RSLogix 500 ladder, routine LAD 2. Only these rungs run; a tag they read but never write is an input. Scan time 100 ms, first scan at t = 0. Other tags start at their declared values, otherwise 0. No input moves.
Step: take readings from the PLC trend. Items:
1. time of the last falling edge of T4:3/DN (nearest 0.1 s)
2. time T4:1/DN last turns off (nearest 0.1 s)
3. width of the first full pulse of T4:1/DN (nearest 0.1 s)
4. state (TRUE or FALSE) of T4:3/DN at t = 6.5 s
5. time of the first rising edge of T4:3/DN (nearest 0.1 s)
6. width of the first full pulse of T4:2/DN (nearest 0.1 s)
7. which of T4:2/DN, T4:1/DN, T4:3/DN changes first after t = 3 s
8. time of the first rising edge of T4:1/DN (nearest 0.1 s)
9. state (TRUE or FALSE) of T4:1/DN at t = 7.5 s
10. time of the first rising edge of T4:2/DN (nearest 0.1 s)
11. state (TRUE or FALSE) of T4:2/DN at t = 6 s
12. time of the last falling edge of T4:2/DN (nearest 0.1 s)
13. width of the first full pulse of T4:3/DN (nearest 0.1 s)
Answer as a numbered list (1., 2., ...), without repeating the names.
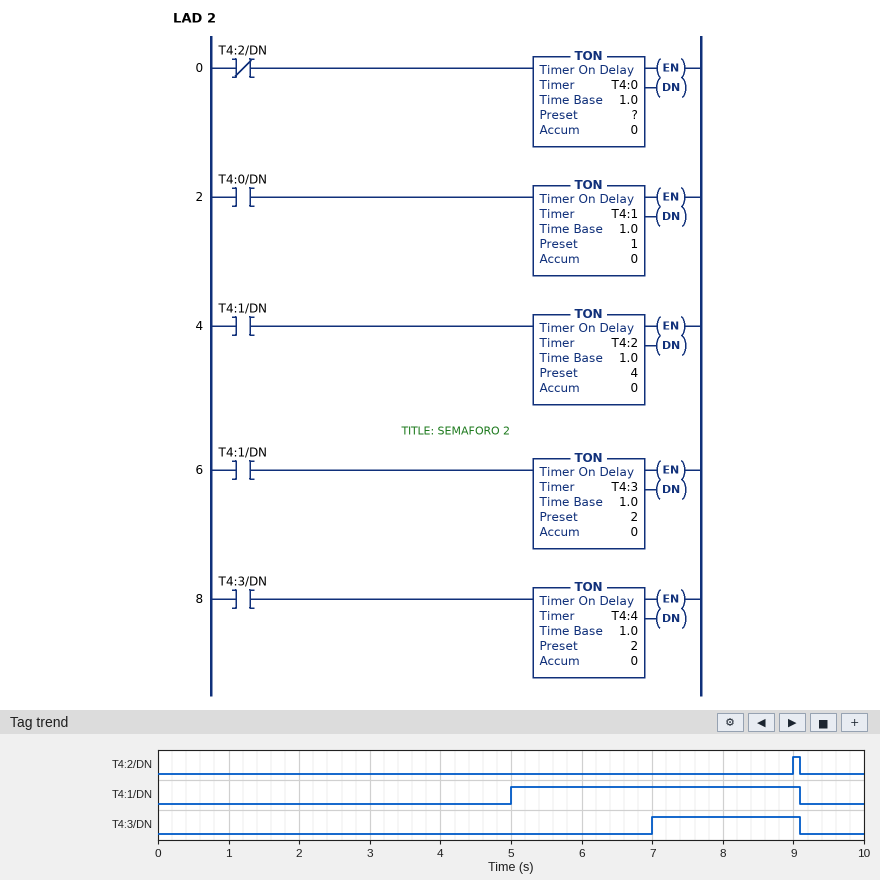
1. 9.1 s
2. 9.1 s
3. 4.1 s
4. FALSE
5. 7.0 s
6. 0.1 s
7. T4:1/DN
8. 5.0 s
9. TRUE
10. 9.0 s
11. FALSE
12. 9.1 s
13. 2.1 s
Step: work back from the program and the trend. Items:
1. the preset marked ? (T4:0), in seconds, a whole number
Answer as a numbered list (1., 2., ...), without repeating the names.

1. 4 s
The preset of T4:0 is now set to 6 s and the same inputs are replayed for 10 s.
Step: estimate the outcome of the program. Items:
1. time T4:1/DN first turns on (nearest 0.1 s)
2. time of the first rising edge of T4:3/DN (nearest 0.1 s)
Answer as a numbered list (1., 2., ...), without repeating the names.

1. 7.0 s
2. 9.0 s
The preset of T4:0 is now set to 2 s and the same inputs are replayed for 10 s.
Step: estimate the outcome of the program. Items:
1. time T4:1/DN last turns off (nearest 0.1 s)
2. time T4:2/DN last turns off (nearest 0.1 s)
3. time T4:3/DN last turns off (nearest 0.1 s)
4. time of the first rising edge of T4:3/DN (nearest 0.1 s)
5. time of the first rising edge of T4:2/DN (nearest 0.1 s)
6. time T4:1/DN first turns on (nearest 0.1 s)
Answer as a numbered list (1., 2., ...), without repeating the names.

1. 7.1 s
2. 7.1 s
3. 7.1 s
4. 5.0 s
5. 7.0 s
6. 3.0 s
